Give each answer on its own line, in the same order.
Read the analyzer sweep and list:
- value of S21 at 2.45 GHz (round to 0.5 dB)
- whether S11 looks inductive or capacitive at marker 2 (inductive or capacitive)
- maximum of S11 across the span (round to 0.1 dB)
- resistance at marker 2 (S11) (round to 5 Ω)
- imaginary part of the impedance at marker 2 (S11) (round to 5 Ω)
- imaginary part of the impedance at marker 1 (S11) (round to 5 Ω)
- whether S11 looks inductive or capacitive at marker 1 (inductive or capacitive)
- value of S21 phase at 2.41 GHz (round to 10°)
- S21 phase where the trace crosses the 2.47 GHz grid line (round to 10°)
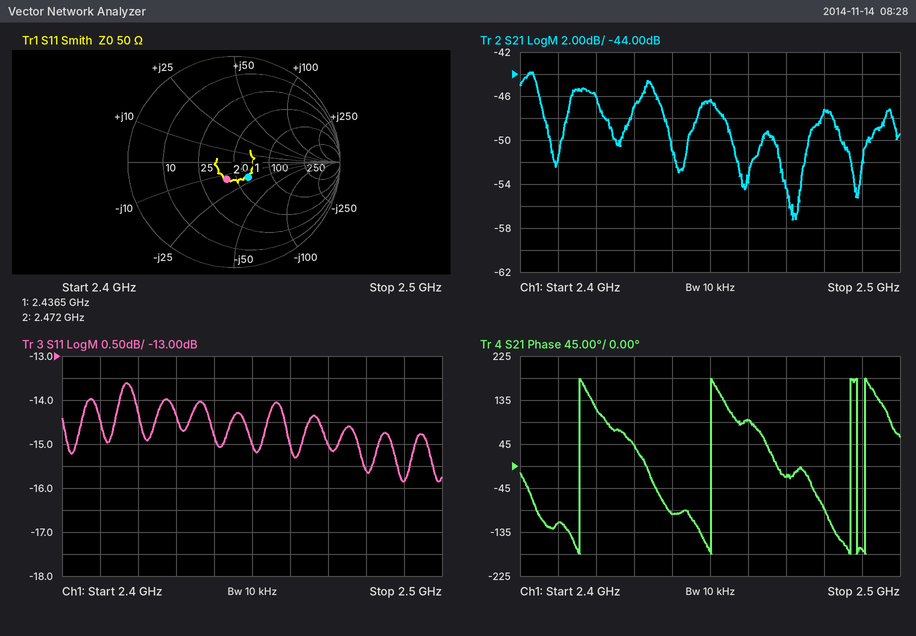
-46.5 dB
capacitive
-13.6 dB
40 Ω
-15 Ω
-20 Ω
capacitive
-120°
-20°
